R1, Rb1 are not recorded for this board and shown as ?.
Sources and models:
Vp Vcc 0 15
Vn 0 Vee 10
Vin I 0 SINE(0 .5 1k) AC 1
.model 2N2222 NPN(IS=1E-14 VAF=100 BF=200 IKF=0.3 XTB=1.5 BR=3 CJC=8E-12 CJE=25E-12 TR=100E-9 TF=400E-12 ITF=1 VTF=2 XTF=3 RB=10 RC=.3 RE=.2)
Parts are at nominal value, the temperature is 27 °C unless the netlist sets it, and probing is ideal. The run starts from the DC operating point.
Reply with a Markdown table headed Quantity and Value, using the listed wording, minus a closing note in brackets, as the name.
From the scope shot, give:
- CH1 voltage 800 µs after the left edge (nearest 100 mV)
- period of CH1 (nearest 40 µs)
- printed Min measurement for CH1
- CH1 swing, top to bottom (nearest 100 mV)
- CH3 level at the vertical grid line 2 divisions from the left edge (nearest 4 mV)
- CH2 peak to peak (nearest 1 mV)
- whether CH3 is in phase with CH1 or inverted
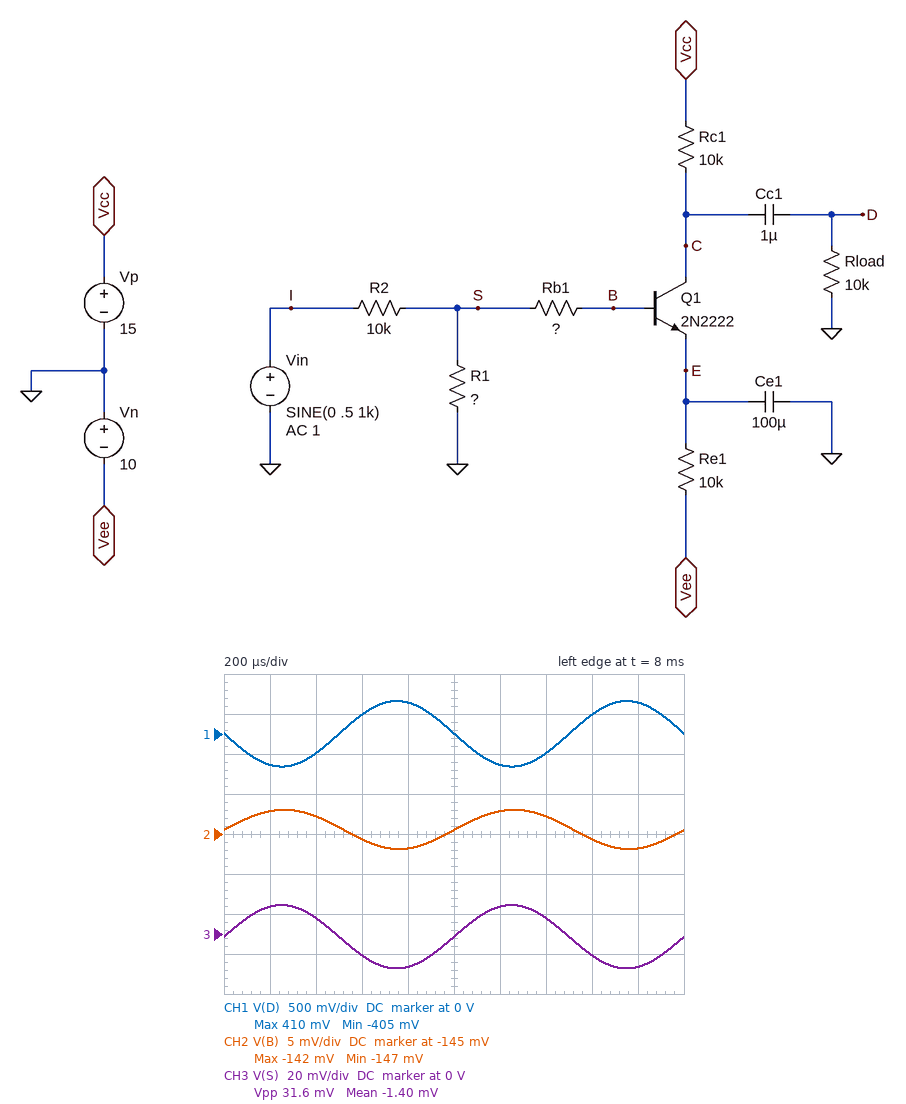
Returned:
| Quantity | Value |
|---|---|
| CH1 voltage 800 µs after the left edge | 400 mV |
| period of CH1 | 1.00 ms |
| printed Min measurement for CH1 | -405 mV |
| CH1 swing, top to bottom | 800 mV |
| CH3 level at the vertical grid line 2 divisions from the left edge | 8 mV |
| CH2 peak to peak | 5 mV |
| whether CH3 is in phase with CH1 or inverted | inverted |
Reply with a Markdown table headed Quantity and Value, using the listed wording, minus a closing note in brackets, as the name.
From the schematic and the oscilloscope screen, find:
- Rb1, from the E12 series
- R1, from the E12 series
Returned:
| Quantity | Value |
|---|---|
| Rb1, from the E12 series | 33 kΩ |
| R1, from the E12 series | 330 Ω |
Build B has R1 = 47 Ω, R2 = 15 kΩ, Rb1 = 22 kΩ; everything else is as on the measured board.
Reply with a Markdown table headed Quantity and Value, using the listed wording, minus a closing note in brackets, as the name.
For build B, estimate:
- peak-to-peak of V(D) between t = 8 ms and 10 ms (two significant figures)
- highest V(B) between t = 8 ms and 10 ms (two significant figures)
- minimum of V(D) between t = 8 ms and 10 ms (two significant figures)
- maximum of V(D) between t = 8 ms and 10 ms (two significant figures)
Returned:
| Quantity | Value |
|---|---|
| peak-to-peak of V(D) between t = 8 ms and 10 ms | 110 mV |
| highest V(B) between t = 8 ms and 10 ms | -96 mV |
| minimum of V(D) between t = 8 ms and 10 ms | -56 mV |
| maximum of V(D) between t = 8 ms and 10 ms | 57 mV |
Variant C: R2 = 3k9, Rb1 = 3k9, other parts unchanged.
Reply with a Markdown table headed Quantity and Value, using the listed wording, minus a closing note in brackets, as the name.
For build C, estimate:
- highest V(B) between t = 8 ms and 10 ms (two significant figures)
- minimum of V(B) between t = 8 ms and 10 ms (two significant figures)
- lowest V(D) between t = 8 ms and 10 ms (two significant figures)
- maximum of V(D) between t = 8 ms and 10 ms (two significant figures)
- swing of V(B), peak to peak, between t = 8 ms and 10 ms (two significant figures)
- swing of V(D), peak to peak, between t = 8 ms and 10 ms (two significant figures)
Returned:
| Quantity | Value |
|---|---|
| highest V(B) between t = 8 ms and 10 ms | 2.8 mV |
| minimum of V(B) between t = 8 ms and 10 ms | -45 mV |
| lowest V(D) between t = 8 ms and 10 ms | -4.0 V |
| maximum of V(D) between t = 8 ms and 10 ms | 3.2 V |
| swing of V(B), peak to peak, between t = 8 ms and 10 ms | 48 mV |
| swing of V(D), peak to peak, between t = 8 ms and 10 ms | 7.2 V |
